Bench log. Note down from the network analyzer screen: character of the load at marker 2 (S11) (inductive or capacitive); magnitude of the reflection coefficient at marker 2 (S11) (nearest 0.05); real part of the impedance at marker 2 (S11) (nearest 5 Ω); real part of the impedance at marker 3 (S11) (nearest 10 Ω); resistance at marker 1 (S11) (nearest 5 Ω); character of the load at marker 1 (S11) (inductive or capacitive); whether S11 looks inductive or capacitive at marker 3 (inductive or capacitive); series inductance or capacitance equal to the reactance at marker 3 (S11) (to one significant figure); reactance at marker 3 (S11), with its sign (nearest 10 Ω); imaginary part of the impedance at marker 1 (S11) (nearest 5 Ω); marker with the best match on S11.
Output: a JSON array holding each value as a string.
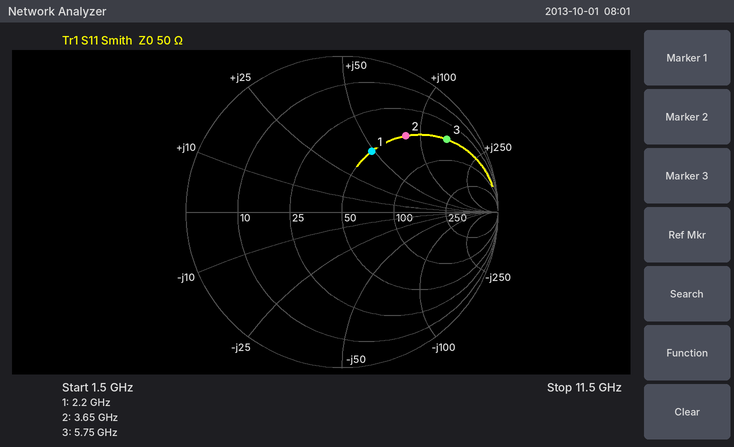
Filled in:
["inductive", "0.65", "50 Ω", "50 Ω", "50 Ω", "inductive", "inductive", "4 nH", "+140 Ω", "+50 Ω", "marker 1"]
